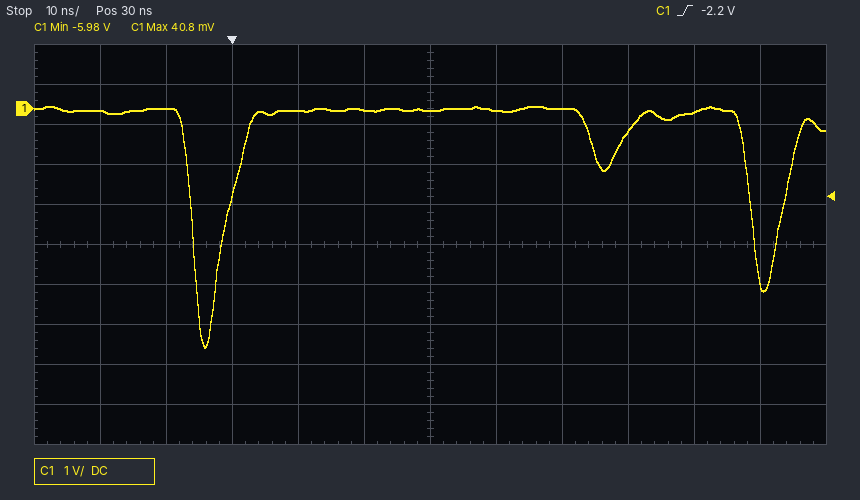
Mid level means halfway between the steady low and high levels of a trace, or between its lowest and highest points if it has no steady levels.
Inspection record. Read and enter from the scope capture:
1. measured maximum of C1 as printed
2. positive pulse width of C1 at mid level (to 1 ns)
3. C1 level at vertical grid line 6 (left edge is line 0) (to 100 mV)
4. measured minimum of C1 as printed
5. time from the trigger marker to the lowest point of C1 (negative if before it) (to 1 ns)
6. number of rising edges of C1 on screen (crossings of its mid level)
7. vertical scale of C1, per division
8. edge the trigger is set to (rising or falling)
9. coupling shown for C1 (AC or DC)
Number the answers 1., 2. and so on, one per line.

1. 40.8 mV
2. 80 ns
3. 0.0 V
4. -5.98 V
5. -4 ns
6. 2
7. 1 V
8. rising
9. DC
